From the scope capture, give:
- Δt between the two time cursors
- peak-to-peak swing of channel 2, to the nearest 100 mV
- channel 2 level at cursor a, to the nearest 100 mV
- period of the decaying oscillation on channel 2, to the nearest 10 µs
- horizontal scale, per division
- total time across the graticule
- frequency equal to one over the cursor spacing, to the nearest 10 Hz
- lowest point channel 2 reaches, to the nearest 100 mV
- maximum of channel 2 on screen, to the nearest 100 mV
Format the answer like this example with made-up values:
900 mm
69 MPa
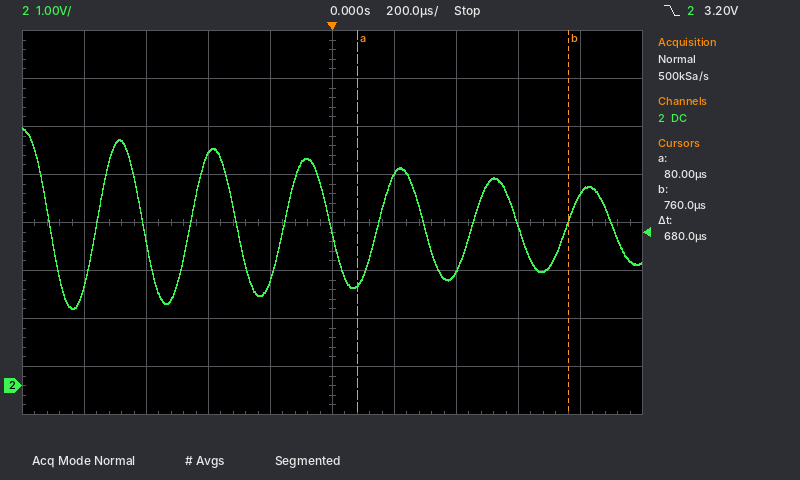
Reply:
680 µs
3.8 V
2.1 V
300 µs
200 µs
2 ms
1.47 kHz
1.6 V
5.4 V
